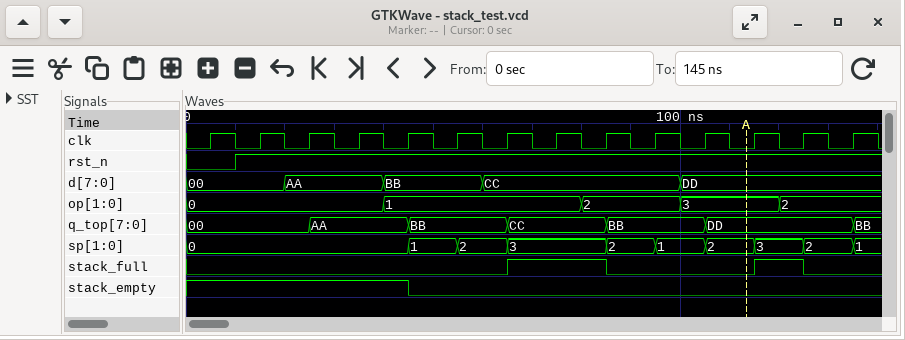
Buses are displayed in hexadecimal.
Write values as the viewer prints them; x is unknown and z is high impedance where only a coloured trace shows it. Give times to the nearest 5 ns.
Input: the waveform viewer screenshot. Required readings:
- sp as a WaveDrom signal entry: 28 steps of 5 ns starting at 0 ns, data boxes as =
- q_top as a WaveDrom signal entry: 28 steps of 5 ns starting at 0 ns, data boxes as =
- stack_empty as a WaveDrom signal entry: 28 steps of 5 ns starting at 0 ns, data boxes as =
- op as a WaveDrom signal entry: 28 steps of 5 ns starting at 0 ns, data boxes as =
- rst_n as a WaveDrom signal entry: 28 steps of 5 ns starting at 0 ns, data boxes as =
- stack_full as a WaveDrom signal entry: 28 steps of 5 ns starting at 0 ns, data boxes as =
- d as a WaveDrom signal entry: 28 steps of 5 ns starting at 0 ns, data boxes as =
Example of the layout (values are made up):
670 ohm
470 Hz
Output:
{name: 'sp', wave: '=........=.=.=...=.=.=.=.=.=', data: '0 1 2 3 2 1 2 3 2 1'}
{name: 'q_top', wave: '=....=...=...=...=...=.....=', data: '00 AA BB CC BB DD BB'}
{name: 'stack_empty', wave: '1........0..................'}
{name: 'op', wave: '=.......=.......=...=...=...', data: '0 1 2 3 2'}
{name: 'rst_n', wave: '0.1.........................'}
{name: 'stack_full', wave: '0............1...0.....1.0..'}
{name: 'd', wave: '=...=...=...=.......=.......', data: '00 AA BB CC DD'}
